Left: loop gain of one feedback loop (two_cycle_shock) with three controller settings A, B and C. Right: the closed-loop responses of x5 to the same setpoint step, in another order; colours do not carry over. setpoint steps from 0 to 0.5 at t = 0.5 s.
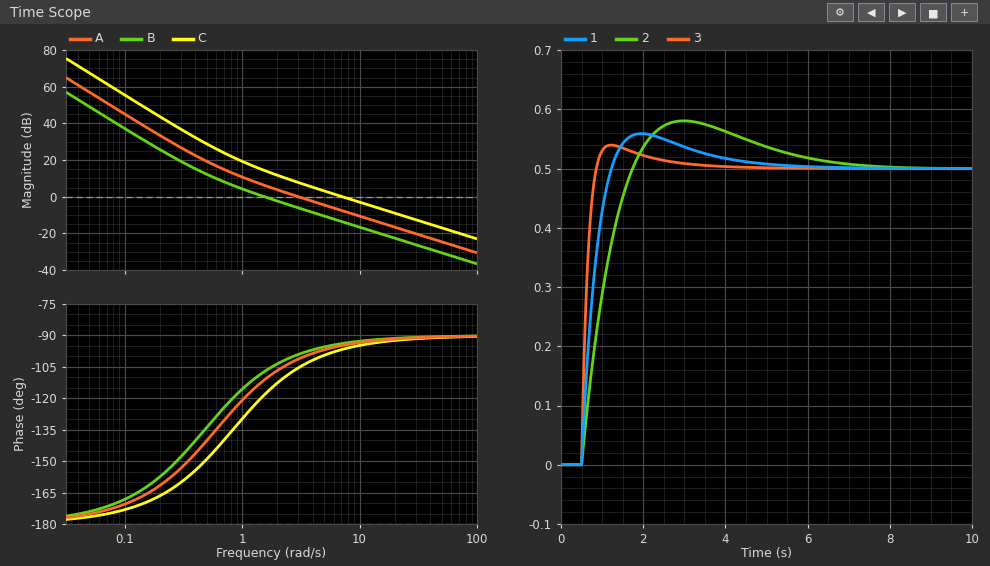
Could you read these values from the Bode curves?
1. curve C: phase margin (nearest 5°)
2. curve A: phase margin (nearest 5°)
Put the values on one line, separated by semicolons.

85°; 80°
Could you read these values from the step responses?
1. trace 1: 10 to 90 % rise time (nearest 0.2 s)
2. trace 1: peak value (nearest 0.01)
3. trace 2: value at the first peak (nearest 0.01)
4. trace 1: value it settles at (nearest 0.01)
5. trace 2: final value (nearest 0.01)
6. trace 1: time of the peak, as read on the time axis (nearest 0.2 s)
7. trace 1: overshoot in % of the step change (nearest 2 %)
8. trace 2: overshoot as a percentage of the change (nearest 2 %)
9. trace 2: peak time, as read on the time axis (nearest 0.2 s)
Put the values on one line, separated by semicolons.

0.6 s; 0.56; 0.58; 0.50; 0.50; 2.0 s; 12 %; 16 %; 3.0 s
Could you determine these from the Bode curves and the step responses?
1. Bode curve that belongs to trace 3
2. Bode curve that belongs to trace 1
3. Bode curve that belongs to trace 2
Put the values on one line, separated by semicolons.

C; A; B
